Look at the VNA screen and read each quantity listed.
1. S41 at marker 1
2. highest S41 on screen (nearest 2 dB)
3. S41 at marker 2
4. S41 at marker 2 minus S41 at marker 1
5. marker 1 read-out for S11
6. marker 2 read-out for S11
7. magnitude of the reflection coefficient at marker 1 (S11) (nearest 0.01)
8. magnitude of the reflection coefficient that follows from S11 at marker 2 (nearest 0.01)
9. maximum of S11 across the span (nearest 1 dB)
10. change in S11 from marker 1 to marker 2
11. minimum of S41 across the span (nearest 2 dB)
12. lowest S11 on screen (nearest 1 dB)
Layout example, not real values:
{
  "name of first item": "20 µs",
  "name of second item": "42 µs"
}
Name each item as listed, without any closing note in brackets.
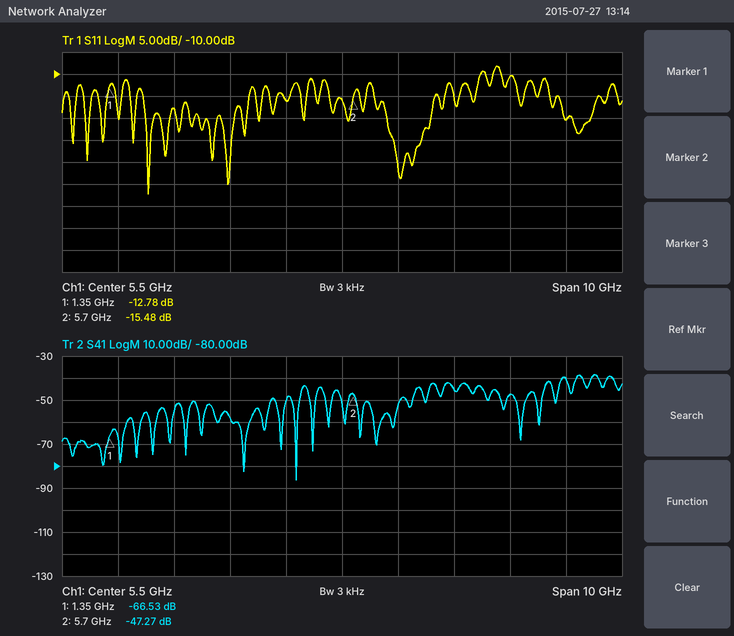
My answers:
{
  "S41 at marker 1": "-66.53 dB",
  "highest S41 on screen": "-38 dB",
  "S41 at marker 2": "-47.27 dB",
  "S41 at marker 2 minus S41 at marker 1": "19.26 dB",
  "marker 1 read-out for S11": "-12.78 dB",
  "marker 2 read-out for S11": "-15.48 dB",
  "magnitude of the reflection coefficient at marker 1 (S11)": "0.23",
  "magnitude of the reflection coefficient that follows from S11 at marker 2": "0.17",
  "maximum of S11 across the span": "-8 dB",
  "change in S11 from marker 1 to marker 2": "-2.70 dB",
  "minimum of S41 across the span": "-86 dB",
  "lowest S11 on screen": "-37 dB"
}
